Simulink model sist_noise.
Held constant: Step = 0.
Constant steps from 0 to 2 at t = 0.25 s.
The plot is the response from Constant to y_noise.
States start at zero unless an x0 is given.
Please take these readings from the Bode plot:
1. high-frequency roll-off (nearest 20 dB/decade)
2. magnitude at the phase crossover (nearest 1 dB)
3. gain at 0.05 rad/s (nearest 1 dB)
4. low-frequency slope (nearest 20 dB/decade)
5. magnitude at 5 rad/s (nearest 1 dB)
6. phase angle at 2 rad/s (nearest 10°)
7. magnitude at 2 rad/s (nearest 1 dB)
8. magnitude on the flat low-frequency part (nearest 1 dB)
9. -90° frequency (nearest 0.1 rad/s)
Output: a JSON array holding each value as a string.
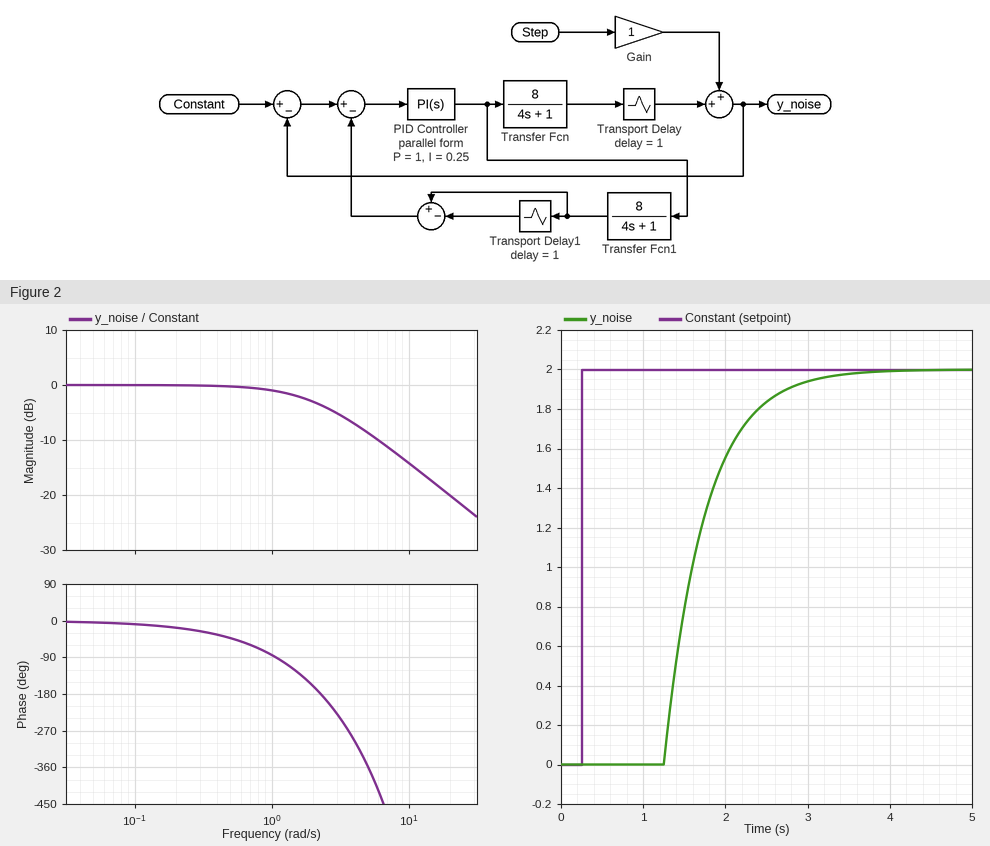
["-20 dB/decade", "-4 dB", "0 dB", "0 dB/decade", "-9 dB", "-160°", "-3 dB", "0 dB", "1.1 rad/s"]
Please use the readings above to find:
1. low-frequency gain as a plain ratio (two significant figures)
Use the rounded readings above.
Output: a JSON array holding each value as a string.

["1.0"]
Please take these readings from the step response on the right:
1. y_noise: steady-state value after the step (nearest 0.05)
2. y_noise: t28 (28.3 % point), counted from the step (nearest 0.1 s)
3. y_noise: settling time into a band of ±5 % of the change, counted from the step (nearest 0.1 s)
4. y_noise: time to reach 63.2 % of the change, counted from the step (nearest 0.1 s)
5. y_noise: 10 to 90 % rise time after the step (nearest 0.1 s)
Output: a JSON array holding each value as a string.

["2.00", "1.2 s", "2.5 s", "1.5 s", "1.1 s"]
